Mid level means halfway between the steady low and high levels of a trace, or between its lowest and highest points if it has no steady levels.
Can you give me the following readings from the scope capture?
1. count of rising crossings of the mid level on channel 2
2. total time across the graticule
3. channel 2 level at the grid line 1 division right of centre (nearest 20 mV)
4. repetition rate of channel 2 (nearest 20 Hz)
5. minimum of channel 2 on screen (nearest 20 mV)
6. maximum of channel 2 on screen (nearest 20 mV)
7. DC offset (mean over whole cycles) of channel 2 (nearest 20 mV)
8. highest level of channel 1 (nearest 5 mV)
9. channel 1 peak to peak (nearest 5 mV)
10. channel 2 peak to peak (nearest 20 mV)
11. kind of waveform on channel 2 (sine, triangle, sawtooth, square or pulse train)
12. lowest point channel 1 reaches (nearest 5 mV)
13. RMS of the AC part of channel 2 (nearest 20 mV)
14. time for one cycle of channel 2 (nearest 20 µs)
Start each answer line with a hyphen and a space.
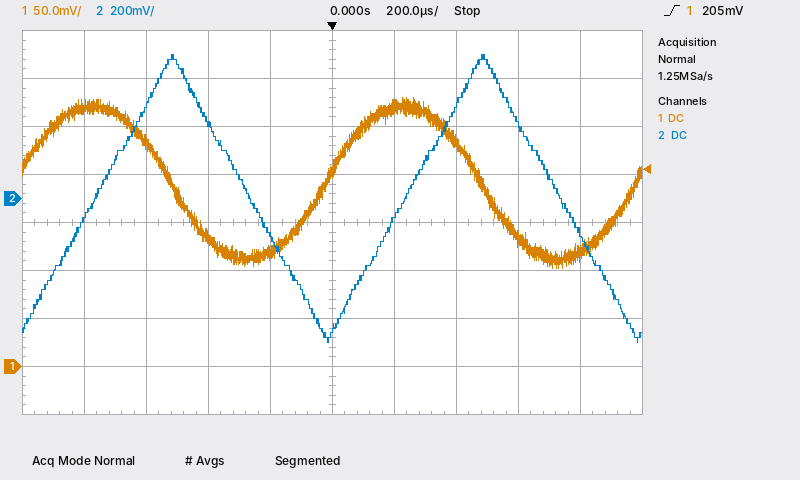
- 2
- 2 ms
- -80 mV
- 1.00 kHz
- -600 mV
- 600 mV
- 0 mV
- 280 mV
- 180 mV
- 1.20 V
- triangle
- 100 mV
- 340 mV
- 1.00 ms
